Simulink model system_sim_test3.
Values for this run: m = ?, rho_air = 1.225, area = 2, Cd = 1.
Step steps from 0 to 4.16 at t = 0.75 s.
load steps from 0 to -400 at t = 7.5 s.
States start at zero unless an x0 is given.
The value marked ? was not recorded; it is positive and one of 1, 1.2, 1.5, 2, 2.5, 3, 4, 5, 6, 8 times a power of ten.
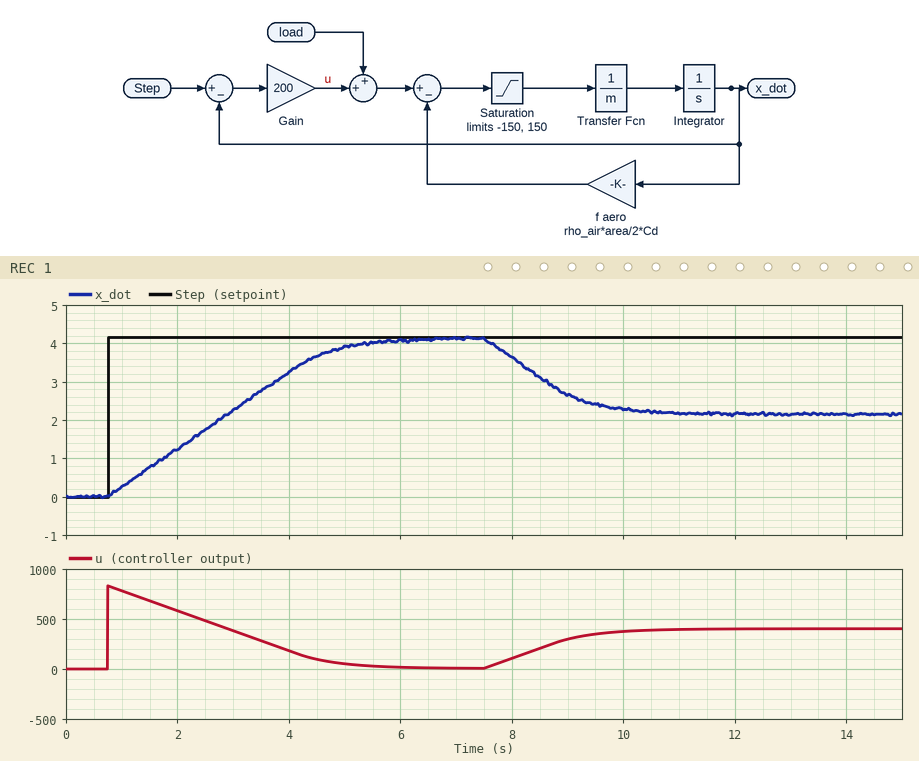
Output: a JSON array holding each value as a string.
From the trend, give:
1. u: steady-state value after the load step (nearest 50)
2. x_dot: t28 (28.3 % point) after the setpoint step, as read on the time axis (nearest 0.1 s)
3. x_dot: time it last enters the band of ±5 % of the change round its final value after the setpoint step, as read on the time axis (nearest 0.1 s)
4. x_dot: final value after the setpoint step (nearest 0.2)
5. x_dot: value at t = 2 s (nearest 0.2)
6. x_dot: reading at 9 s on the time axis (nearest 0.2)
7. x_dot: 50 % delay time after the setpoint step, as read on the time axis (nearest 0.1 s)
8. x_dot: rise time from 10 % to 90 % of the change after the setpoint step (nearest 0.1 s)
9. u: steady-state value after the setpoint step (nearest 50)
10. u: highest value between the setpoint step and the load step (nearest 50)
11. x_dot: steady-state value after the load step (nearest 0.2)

["400", "1.9 s", "5.1 s", "4.2", "1.2", "2.6", "2.8 s", "3.4 s", "0", "850", "2.2"]
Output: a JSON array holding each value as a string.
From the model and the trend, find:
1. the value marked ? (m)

["150"]
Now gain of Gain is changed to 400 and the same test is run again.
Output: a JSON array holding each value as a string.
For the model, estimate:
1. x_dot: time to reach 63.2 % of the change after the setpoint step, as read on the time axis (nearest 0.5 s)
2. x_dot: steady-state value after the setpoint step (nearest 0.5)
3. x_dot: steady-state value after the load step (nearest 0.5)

["3.5 s", "4.0", "3.0"]
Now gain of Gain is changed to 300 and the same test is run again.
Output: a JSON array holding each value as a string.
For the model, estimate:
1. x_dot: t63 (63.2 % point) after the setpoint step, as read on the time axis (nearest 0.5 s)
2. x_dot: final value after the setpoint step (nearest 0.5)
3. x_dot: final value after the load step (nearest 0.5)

["3.5 s", "4.0", "3.0"]
